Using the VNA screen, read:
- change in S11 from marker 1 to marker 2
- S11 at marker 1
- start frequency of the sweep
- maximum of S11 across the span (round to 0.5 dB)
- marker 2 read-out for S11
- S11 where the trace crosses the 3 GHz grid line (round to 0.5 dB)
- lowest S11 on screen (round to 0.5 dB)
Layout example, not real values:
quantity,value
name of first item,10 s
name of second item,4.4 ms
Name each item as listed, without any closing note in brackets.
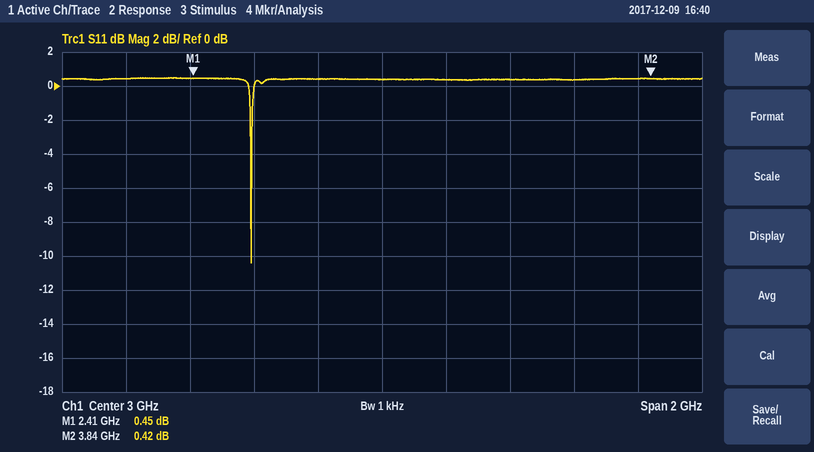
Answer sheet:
quantity,value
change in S11 from marker 1 to marker 2,-0.03 dB
S11 at marker 1,0.45 dB
start frequency of the sweep,2 GHz
maximum of S11 across the span,0.5 dB
marker 2 read-out for S11,0.42 dB
S11 where the trace crosses the 3 GHz grid line,0.5 dB
lowest S11 on screen,-10.5 dB
